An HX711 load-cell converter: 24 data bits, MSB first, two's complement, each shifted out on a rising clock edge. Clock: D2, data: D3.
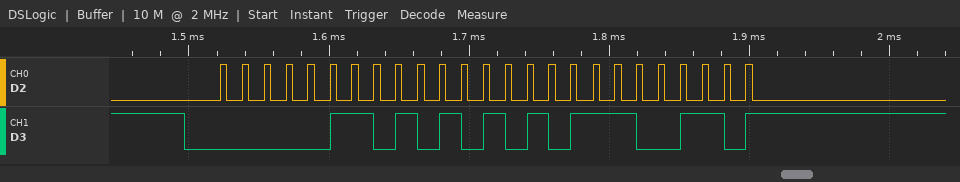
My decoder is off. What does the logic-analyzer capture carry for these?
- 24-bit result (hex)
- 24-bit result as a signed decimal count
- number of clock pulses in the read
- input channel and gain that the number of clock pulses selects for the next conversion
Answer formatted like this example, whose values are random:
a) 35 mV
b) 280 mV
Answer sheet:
a) 0x06AAE6
b) 436966
c) 25
d) channel A, gain 128
